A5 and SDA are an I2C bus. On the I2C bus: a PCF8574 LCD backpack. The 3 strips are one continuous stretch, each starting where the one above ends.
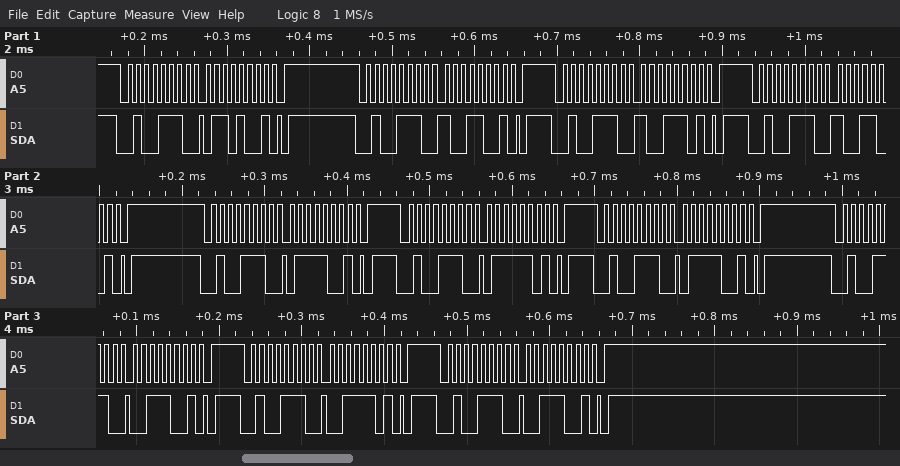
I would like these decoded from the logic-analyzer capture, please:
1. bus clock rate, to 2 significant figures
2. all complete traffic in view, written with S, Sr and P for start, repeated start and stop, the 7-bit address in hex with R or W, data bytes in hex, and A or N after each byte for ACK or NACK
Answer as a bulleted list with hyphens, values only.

- 100 kHz
- S 27W A 69 A P S 27W A 99 A P S 27W A 9D A P S 27W A 99 A P S 27W A 79 A P S 27W A 7D A P S 27W A 79 A P S 27W A 39 A P S 27W A 3D A P S 27W A 39 A P
